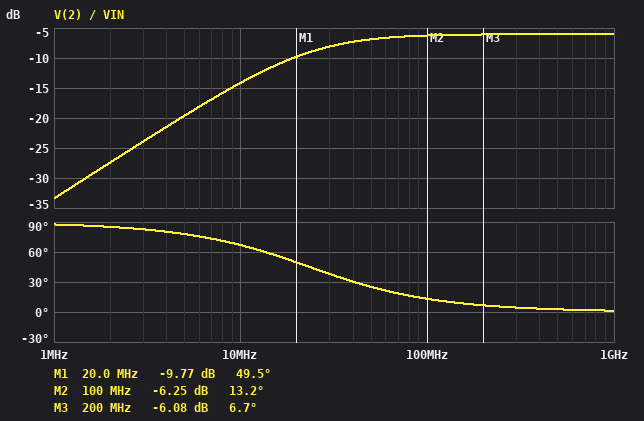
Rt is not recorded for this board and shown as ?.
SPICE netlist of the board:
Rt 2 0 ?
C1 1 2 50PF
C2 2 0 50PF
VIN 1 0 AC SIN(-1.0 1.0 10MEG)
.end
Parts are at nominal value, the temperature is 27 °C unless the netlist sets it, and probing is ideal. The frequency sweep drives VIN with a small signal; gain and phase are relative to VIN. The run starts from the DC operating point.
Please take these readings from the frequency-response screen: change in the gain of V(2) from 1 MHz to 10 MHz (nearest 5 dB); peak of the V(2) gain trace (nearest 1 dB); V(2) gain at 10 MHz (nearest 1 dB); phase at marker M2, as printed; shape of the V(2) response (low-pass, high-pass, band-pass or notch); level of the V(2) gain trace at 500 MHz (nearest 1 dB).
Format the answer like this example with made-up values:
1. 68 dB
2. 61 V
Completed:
1. 20 dB
2. -6 dB
3. -14 dB
4. 13.2 deg
5. high-pass
6. -6 dB
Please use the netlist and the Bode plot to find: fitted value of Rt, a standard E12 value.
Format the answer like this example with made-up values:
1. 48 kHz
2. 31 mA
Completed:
1. 68 Ω
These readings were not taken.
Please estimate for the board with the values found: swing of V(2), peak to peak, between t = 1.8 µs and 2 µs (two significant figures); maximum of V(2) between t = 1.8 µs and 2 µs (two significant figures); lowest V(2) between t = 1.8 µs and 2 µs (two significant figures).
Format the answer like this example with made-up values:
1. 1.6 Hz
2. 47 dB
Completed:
1. 390 mV
2. 200 mV
3. -200 mV
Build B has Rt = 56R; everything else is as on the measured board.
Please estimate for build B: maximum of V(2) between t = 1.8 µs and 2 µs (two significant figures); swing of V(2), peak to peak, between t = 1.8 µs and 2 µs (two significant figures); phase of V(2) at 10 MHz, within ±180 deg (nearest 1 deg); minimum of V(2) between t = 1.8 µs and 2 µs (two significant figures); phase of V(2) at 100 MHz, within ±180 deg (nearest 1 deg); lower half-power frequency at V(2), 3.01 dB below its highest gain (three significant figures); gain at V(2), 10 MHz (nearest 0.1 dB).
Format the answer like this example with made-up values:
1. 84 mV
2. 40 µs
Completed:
1. 170 mV
2. 330 mV
3. 71 deg
4. -170 mV
5. 16 deg
6. 28.4 MHz
7. -15.6 dB
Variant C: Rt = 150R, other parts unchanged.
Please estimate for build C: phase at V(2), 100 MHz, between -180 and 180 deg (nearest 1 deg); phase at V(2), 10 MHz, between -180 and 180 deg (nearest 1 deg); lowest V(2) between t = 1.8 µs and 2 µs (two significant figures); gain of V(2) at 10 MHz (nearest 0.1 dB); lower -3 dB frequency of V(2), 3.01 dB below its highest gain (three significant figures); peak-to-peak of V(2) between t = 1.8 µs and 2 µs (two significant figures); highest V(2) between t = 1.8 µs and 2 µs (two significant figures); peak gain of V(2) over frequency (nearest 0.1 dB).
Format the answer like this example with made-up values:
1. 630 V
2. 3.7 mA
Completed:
1. 6 deg
2. 47 deg
3. -340 mV
4. -9.3 dB
5. 10.6 MHz
6. 690 mV
7. 340 mV
8. -6.0 dB
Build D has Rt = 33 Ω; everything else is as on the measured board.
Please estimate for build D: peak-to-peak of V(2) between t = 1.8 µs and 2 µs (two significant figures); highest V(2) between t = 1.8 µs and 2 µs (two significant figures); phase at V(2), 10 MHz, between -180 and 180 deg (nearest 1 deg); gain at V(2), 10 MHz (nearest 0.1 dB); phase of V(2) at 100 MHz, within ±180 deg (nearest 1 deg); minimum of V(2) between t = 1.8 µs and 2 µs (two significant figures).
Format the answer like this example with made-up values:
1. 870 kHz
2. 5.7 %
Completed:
1. 200 mV
2. 100 mV
3. 78 deg
4. -19.9 dB
5. 26 deg
6. -100 mV
